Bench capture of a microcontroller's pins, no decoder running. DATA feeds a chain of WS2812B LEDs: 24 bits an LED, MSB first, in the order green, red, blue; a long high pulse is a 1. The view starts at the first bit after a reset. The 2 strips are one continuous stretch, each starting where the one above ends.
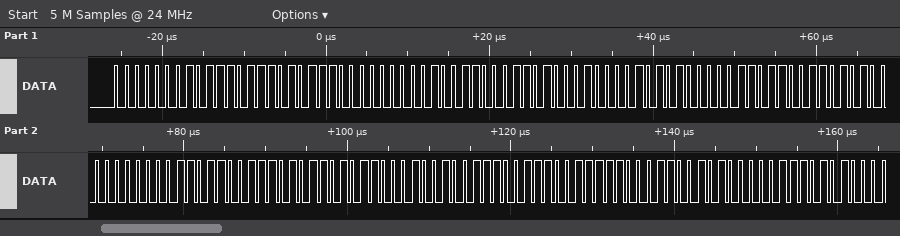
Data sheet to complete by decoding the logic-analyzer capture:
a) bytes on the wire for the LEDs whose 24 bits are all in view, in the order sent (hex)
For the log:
01 77 5C 01 31 A2 15 06 CD 40 0D 9D 6B 12 73 9F 19 41
